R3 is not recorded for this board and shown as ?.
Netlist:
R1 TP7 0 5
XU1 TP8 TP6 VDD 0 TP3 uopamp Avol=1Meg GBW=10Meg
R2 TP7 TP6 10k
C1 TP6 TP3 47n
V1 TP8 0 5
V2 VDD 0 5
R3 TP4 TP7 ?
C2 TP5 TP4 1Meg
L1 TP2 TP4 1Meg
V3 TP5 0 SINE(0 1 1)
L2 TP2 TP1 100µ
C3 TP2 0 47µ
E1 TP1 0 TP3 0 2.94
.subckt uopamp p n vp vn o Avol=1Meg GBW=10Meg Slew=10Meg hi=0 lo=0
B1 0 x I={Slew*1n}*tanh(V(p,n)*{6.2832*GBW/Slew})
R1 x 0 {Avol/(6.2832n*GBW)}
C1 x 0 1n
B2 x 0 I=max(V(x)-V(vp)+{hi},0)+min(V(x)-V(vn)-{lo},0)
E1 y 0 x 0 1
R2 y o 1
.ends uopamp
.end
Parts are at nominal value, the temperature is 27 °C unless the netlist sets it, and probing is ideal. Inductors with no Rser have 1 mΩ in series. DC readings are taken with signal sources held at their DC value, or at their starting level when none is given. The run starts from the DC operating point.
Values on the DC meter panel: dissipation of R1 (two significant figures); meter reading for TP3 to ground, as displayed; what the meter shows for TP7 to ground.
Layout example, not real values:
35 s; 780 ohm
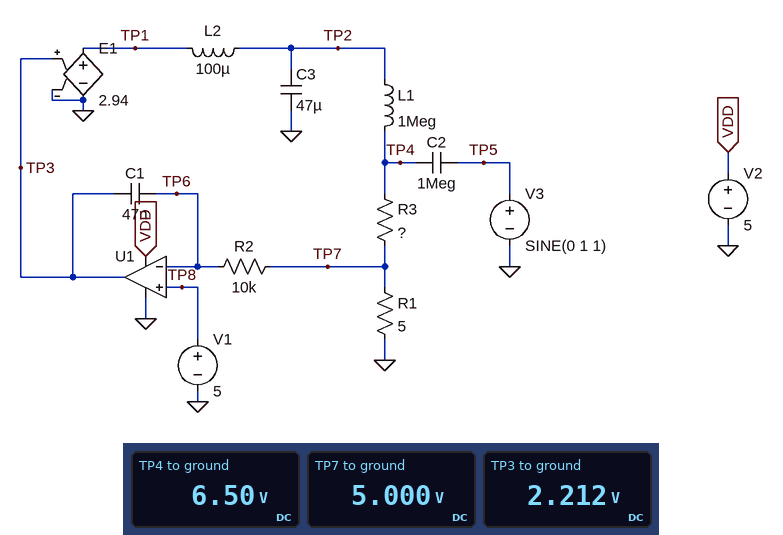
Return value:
5.0 W; 2.212 V; 5.000 V
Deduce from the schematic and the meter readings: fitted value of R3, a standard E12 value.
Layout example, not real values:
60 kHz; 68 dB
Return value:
1.5 Ω
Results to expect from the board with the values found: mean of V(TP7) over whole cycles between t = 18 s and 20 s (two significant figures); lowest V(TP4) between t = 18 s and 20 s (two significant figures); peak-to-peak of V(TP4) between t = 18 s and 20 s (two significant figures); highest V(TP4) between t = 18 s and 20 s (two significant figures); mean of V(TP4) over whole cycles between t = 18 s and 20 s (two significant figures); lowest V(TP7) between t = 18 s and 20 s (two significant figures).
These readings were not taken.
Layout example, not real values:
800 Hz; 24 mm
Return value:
5.0 V; 5.5 V; 2.0 V; 7.5 V; 6.5 V; 4.2 V
